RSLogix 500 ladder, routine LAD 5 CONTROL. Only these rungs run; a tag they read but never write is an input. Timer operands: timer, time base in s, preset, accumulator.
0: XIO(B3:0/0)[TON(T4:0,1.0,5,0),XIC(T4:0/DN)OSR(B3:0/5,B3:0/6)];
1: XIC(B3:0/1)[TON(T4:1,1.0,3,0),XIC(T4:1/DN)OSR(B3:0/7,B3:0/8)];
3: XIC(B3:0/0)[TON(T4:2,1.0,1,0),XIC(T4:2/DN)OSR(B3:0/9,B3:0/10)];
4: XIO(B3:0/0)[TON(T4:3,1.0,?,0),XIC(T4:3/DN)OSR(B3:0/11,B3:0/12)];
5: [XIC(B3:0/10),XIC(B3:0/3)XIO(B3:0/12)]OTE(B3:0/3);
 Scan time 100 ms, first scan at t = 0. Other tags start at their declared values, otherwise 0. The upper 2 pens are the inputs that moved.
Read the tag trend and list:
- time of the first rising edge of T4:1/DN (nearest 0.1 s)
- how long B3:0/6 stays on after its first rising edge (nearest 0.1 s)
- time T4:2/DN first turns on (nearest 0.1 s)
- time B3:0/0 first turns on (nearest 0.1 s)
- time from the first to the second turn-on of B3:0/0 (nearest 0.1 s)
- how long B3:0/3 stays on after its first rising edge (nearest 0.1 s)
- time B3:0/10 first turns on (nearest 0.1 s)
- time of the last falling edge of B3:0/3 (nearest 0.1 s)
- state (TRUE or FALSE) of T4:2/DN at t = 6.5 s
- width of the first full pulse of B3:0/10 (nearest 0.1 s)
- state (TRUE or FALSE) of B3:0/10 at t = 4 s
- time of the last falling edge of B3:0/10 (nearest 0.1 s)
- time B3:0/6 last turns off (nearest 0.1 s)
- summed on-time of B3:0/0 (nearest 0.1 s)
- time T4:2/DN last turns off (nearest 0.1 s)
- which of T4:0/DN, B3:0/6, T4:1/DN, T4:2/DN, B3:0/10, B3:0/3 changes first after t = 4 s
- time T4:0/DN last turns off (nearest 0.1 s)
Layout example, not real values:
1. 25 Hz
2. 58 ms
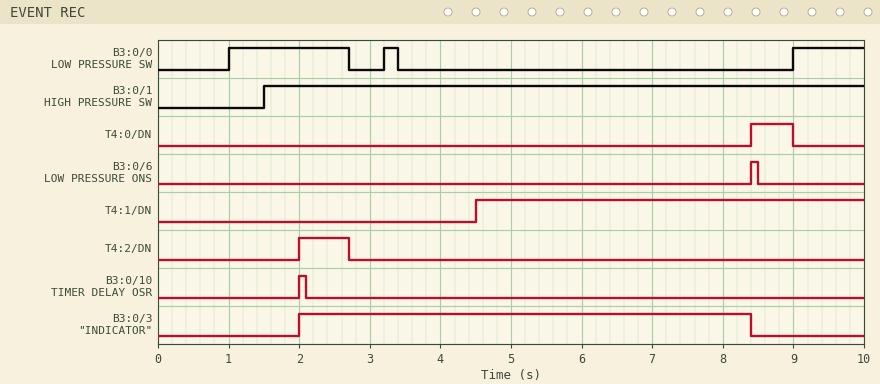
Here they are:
1. 4.5 s
2. 0.1 s
3. 2.0 s
4. 1.0 s
5. 2.2 s
6. 6.4 s
7. 2.0 s
8. 8.4 s
9. FALSE
10. 0.1 s
11. FALSE
12. 2.1 s
13. 8.5 s
14. 2.9 s
15. 2.7 s
16. T4:1/DN
17. 9.0 s
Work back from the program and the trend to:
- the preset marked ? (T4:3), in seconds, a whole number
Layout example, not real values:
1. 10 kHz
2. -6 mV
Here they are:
1. 5 s
